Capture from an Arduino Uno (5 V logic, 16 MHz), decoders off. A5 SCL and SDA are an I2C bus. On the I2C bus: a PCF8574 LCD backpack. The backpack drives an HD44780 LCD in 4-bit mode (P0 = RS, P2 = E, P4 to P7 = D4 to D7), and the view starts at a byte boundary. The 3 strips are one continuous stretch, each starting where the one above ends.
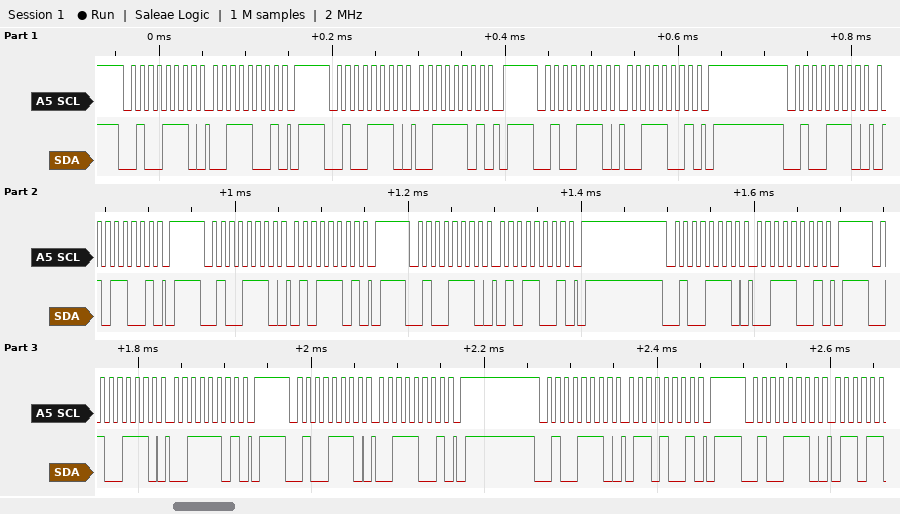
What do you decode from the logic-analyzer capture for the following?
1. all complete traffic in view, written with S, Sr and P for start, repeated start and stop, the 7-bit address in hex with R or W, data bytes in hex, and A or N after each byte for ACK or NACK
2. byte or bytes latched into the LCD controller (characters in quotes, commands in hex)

S 27W A 39 A P S 27W A 3D A P S 27W A 39 A P S 27W A 59 A P S 27W A 5D A P S 27W A 59 A P S 27W A 39 A P S 27W A 3D A P S 27W A 39 A P S 27W A 69 A P S 27W A
'5'
